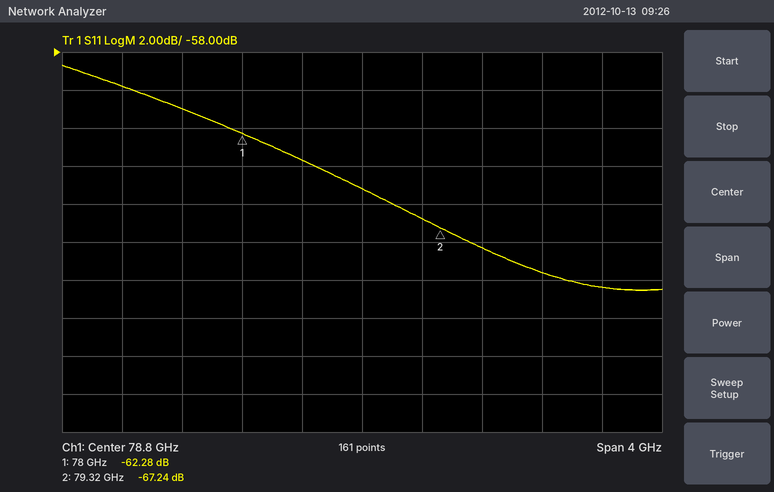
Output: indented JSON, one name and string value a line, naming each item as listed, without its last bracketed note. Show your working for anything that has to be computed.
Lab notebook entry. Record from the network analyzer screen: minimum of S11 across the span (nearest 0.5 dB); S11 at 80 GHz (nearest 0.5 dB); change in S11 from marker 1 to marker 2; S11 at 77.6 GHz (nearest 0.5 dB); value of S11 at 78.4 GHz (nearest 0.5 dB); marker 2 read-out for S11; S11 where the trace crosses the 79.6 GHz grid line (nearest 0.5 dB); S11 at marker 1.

{
  "minimum of S11 across the span": "-70.5 dB",
  "S11 at 80 GHz": "-69.5 dB",
  "change in S11 from marker 1 to marker 2": "-67.24 − (-62.28) = -4.96 dB",
  "S11 at 77.6 GHz": "-61.0 dB",
  "value of S11 at 78.4 GHz": "-63.5 dB",
  "marker 2 read-out for S11": "-67.24 dB",
  "S11 where the trace crosses the 79.6 GHz grid line": "-68.5 dB",
  "S11 at marker 1": "-62.28 dB"
}
